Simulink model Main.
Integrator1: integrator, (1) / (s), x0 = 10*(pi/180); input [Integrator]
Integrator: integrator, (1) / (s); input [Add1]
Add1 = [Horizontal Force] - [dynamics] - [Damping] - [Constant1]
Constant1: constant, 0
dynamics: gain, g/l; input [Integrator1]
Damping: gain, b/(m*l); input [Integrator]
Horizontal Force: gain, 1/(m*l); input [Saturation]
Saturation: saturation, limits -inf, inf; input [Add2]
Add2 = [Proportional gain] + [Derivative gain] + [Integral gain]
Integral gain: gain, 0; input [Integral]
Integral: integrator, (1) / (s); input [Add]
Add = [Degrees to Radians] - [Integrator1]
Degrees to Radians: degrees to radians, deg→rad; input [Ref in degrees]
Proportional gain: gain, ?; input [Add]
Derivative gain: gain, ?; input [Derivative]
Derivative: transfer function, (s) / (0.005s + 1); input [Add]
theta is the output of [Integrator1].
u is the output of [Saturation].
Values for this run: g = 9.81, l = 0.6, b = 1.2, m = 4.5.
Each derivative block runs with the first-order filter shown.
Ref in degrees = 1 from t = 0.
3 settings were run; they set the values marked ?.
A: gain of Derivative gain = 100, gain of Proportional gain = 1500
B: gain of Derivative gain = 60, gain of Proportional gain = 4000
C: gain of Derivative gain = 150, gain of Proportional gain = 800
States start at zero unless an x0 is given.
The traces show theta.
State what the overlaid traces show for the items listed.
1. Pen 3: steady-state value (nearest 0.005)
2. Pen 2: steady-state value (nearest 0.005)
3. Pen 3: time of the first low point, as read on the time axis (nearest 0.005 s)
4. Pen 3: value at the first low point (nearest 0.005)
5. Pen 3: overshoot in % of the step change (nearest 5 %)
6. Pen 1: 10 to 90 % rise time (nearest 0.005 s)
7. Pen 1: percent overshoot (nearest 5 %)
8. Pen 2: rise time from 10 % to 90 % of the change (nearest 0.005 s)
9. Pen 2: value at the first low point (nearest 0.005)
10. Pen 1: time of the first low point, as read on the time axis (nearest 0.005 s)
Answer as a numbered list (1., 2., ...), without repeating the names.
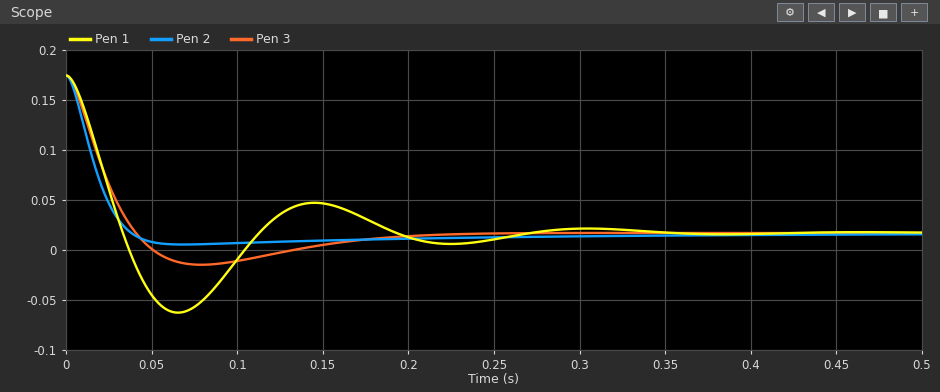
1. 0.015
2. 0.015
3. 0.080 s
4. -0.015
5. 20 %
6. 0.025 s
7. 50 %
8. 0.025 s
9. 0.005
10. 0.065 s
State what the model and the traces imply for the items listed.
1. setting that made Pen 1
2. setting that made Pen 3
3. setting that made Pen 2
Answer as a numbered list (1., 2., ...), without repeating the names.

1. B
2. A
3. C
